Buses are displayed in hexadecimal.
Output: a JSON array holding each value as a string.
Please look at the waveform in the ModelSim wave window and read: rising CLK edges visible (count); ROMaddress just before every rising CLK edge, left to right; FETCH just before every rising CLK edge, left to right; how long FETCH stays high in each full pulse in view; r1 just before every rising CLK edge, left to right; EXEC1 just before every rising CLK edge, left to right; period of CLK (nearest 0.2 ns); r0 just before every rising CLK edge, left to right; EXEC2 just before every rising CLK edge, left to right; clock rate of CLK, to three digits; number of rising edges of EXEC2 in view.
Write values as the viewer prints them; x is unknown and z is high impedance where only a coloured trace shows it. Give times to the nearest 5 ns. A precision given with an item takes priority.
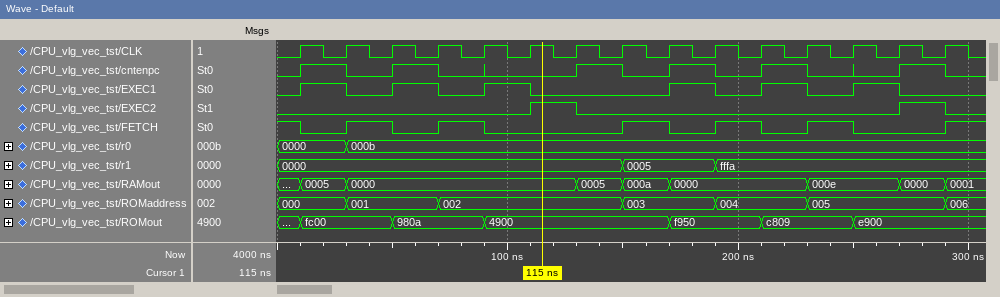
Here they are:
["15", "000, 000, 001, 001, 002, 002, 002, 002, 003, 003, 004, 004, 005, 005, 005", "1 0 1 0 1 0 0 0 1 0 1 0 1 0 0", "20 ns, 20 ns, 20 ns, 20 ns, 20 ns", "0000, 0000, 0000, 0000, 0000, 0000, 0000, 0000, 0005, 0005, fffa, fffa, fffa, fffa, fffa", "0 1 0 1 0 1 0 0 0 1 0 1 0 1 0", "20 ns", "0000, 0000, 000b, 000b, 000b, 000b, 000b, 000b, 000b, 000b, 000b, 000b, 000b, 000b, 000b", "0 0 0 0 0 0 1 0 0 0 0 0 0 0 1", "50.0 MHz", "2"]
